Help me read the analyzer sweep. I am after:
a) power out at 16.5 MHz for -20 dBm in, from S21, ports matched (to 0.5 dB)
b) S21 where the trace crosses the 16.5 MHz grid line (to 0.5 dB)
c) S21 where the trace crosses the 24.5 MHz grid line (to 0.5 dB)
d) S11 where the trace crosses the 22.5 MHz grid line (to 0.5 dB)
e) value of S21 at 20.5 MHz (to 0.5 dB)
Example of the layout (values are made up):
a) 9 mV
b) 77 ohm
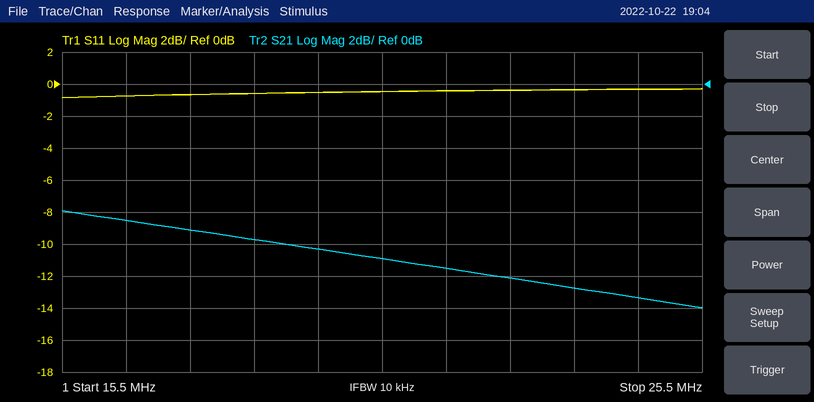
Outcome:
a) -28.5 dBm
b) -8.5 dB
c) -13.5 dB
d) -0.5 dB
e) -11.0 dB
